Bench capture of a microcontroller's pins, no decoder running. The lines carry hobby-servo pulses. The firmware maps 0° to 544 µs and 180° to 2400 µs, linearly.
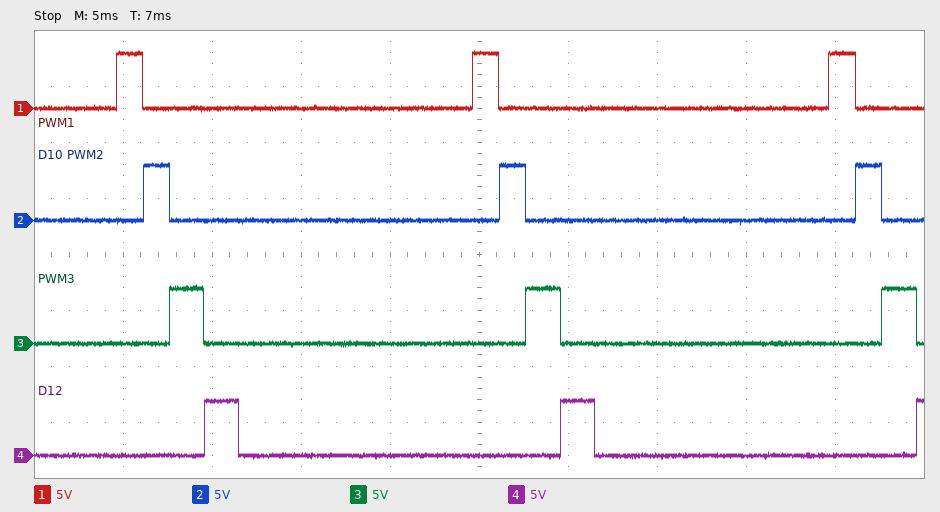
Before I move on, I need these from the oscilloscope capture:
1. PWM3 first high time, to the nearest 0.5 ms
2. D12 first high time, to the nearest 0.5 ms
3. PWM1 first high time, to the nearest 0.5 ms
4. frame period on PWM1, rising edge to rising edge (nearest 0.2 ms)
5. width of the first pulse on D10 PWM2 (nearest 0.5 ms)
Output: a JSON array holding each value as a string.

["2.0 ms", "2.0 ms", "1.5 ms", "20.0 ms", "1.5 ms"]
